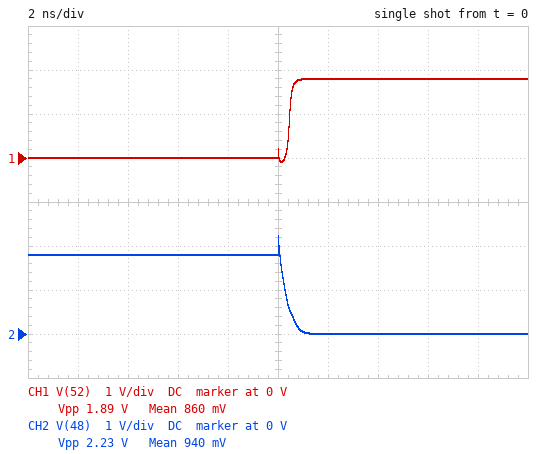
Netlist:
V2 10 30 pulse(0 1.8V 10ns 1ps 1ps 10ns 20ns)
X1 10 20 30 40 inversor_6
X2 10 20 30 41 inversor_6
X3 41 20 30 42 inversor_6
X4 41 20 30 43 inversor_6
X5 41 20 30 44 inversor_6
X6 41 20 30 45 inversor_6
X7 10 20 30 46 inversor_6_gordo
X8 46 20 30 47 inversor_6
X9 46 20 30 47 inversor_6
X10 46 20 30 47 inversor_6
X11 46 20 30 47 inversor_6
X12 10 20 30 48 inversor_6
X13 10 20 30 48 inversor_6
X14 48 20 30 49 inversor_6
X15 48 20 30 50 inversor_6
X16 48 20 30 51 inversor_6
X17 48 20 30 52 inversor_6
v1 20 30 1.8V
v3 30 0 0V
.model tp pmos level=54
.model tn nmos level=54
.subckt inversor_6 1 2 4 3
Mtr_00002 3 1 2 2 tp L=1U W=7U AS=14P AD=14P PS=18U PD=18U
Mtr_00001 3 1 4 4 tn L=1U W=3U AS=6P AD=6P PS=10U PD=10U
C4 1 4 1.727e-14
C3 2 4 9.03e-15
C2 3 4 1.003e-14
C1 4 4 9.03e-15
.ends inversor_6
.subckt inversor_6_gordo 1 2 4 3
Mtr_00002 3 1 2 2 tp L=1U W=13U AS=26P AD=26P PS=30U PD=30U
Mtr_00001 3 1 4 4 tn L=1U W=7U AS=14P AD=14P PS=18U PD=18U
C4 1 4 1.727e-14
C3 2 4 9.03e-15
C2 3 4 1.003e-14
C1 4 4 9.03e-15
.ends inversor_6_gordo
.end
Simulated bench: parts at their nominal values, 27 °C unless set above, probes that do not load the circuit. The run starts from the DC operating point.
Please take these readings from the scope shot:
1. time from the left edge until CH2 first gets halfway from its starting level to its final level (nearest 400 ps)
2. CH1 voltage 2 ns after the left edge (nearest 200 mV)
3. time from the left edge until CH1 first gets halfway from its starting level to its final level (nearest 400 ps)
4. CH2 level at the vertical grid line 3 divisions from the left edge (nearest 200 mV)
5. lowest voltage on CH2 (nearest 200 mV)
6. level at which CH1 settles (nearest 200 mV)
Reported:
10.4 ns
0 V
10.4 ns
1.8 V
0 V
1.8 V
